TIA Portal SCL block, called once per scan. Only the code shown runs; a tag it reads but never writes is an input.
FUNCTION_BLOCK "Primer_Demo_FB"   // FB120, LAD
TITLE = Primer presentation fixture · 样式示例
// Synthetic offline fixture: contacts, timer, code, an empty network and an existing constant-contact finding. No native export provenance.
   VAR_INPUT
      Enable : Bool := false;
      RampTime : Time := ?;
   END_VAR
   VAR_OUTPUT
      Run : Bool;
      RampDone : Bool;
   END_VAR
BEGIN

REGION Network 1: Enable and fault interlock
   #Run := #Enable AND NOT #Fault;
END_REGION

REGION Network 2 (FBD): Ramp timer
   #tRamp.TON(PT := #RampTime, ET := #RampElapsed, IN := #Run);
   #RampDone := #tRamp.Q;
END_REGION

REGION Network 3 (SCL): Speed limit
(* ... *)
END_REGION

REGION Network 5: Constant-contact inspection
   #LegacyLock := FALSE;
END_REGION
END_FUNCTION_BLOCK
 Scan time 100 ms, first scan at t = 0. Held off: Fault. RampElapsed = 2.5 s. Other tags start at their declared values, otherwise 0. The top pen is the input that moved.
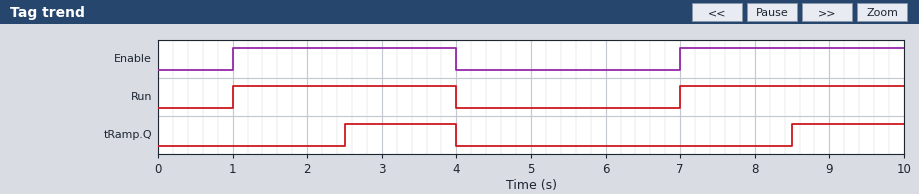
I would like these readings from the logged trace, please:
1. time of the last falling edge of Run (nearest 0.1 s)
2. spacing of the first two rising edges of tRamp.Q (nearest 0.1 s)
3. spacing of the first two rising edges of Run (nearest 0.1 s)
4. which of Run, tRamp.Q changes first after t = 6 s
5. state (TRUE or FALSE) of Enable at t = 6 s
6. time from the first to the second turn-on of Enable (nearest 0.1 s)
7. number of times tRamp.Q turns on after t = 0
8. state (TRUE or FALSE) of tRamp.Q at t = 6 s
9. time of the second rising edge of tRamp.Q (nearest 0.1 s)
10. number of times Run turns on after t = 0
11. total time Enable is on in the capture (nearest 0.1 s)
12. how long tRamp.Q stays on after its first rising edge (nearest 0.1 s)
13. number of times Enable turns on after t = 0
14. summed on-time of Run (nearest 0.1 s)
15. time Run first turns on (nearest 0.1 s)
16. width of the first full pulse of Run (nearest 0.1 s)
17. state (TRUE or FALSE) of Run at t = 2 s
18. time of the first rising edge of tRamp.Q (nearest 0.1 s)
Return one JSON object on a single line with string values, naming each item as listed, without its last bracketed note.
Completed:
{"time of the last falling edge of Run": "4.0 s", "spacing of the first two rising edges of tRamp.Q": "6.0 s", "spacing of the first two rising edges of Run": "6.0 s", "which of Run, tRamp.Q changes first after t = 6 s": "Run", "state (TRUE or FALSE) of Enable at t = 6 s": "FALSE", "time from the first to the second turn-on of Enable": "6.0 s", "number of times tRamp.Q turns on after t = 0": "2", "state (TRUE or FALSE) of tRamp.Q at t = 6 s": "FALSE", "time of the second rising edge of tRamp.Q": "8.5 s", "number of times Run turns on after t = 0": "2", "total time Enable is on in the capture": "6.0 s", "how long tRamp.Q stays on after its first rising edge": "1.5 s", "number of times Enable turns on after t = 0": "2", "summed on-time of Run": "6.0 s", "time Run first turns on": "1.0 s", "width of the first full pulse of Run": "3.0 s", "state (TRUE or FALSE) of Run at t = 2 s": "TRUE", "time of the first rising edge of tRamp.Q": "2.5 s"}
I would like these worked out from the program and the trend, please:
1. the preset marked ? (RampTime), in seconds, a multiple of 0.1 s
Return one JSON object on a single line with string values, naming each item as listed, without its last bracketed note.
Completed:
{"the preset marked ? (RampTime), in seconds, a multiple of 0.1 s": "1.5 s"}
